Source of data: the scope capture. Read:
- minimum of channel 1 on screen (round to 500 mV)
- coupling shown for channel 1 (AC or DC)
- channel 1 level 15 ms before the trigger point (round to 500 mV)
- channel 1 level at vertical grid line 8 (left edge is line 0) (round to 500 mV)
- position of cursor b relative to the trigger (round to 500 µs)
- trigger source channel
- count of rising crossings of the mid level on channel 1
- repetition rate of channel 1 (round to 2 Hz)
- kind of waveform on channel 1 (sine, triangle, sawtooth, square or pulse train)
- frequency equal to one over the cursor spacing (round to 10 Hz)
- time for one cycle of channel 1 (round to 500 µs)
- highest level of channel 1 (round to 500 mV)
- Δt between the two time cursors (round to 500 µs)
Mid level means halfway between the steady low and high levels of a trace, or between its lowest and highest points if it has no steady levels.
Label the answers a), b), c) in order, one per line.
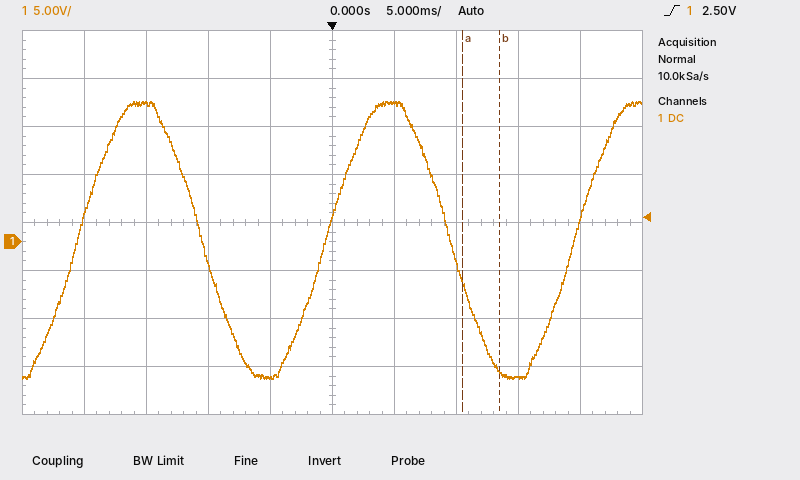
a) -14.0 V
b) DC
c) 14.5 V
d) -14.0 V
e) +13.5 ms
f) channel 1
g) 3
h) 50 Hz
i) sine
j) 330 Hz
k) 20.0 ms
l) 14.5 V
m) 3.0 ms
